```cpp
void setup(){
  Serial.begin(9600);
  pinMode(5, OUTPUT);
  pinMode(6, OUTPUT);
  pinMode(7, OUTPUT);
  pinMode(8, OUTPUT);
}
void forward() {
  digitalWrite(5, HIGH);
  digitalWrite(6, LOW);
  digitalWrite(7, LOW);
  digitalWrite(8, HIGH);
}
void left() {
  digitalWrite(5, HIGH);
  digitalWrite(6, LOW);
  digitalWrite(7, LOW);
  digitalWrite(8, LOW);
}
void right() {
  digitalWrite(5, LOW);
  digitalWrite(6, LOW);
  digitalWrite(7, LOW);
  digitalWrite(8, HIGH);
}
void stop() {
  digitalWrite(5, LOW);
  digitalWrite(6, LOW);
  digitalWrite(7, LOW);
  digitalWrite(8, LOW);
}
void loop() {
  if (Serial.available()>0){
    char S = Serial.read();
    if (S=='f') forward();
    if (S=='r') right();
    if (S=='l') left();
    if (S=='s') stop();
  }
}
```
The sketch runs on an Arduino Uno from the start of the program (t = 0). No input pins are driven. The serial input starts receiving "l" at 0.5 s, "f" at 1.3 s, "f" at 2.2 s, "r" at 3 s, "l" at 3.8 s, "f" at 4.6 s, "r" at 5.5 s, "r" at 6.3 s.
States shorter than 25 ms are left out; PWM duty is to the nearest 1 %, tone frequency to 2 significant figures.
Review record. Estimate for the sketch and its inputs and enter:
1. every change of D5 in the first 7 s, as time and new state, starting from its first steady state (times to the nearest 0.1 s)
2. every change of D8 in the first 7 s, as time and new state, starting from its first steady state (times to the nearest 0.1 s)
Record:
0 s low; 0.5 s high; 3 s low; 3.8 s high; 5.5 s low
0 s low; 1.3 s high; 3.8 s low; 4.6 s high
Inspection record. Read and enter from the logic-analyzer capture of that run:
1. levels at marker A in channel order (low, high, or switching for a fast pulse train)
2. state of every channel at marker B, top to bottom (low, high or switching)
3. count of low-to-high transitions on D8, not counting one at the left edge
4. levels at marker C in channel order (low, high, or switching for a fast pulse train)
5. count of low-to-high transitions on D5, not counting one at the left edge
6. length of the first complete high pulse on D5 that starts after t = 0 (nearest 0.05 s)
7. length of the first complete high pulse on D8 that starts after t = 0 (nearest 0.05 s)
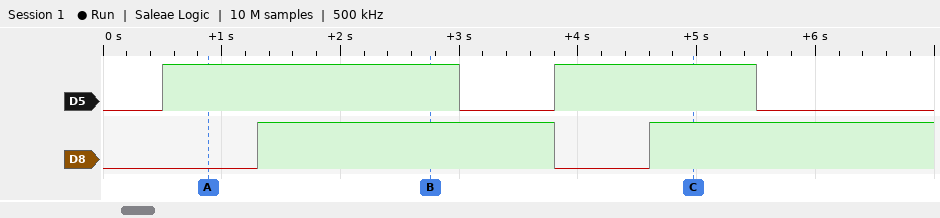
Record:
D5 high, D8 low
D5 high, D8 high
2
D5 high, D8 high
2
2.50 s
2.50 s
